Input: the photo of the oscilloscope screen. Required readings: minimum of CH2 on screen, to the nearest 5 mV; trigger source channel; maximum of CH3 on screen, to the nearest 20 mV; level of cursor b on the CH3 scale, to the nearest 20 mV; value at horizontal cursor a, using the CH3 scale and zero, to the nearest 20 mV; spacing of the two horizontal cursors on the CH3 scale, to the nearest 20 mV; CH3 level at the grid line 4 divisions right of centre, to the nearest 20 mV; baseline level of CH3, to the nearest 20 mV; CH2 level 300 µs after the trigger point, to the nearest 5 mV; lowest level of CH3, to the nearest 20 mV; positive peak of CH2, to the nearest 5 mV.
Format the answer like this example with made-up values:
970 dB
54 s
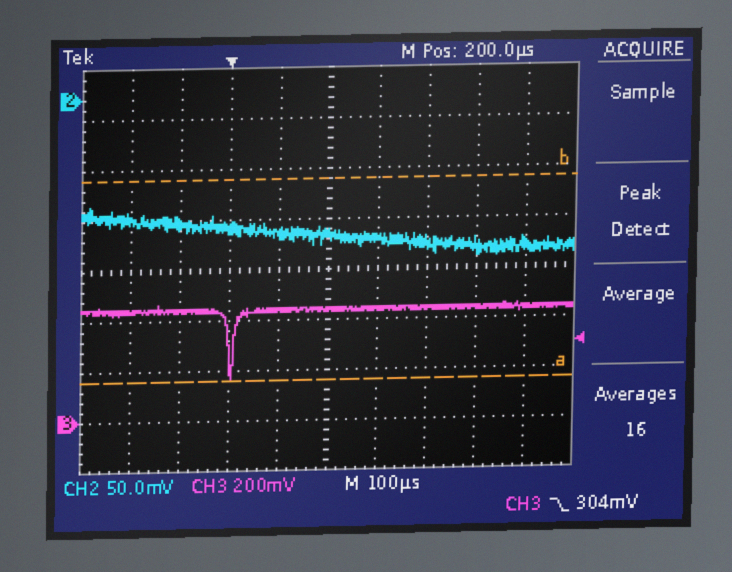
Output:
-160 mV
CH3
460 mV
960 mV
160 mV
800 mV
440 mV
440 mV
-140 mV
160 mV
-105 mV
